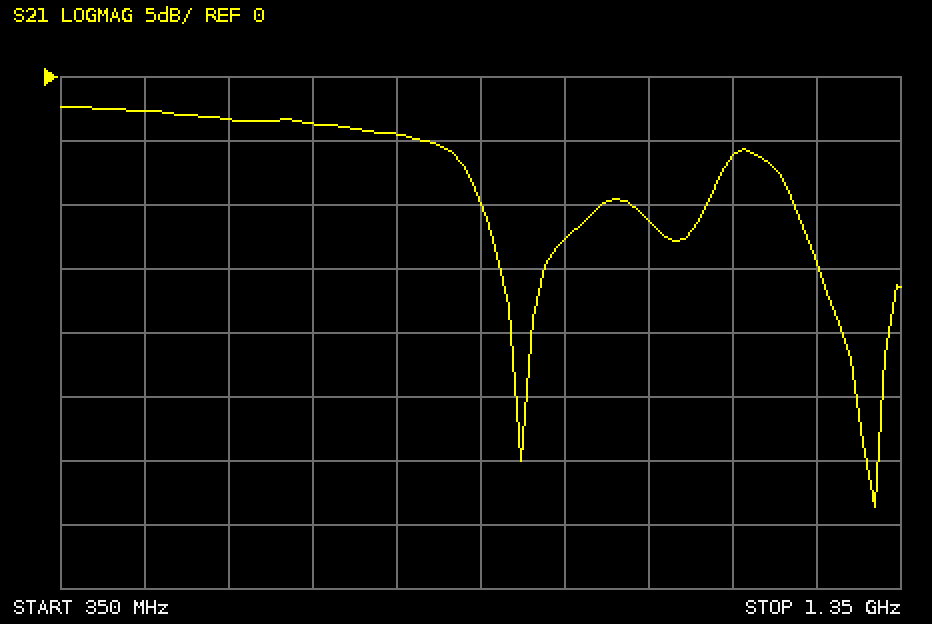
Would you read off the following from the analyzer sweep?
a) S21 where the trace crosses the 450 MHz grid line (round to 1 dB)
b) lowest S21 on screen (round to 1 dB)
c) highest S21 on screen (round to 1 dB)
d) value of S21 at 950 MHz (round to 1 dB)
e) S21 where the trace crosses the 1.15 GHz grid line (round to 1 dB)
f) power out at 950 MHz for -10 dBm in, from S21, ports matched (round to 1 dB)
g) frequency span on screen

-3 dB
-34 dB
-2 dB
-13 dB
-6 dB
-23 dBm
1 GHz
